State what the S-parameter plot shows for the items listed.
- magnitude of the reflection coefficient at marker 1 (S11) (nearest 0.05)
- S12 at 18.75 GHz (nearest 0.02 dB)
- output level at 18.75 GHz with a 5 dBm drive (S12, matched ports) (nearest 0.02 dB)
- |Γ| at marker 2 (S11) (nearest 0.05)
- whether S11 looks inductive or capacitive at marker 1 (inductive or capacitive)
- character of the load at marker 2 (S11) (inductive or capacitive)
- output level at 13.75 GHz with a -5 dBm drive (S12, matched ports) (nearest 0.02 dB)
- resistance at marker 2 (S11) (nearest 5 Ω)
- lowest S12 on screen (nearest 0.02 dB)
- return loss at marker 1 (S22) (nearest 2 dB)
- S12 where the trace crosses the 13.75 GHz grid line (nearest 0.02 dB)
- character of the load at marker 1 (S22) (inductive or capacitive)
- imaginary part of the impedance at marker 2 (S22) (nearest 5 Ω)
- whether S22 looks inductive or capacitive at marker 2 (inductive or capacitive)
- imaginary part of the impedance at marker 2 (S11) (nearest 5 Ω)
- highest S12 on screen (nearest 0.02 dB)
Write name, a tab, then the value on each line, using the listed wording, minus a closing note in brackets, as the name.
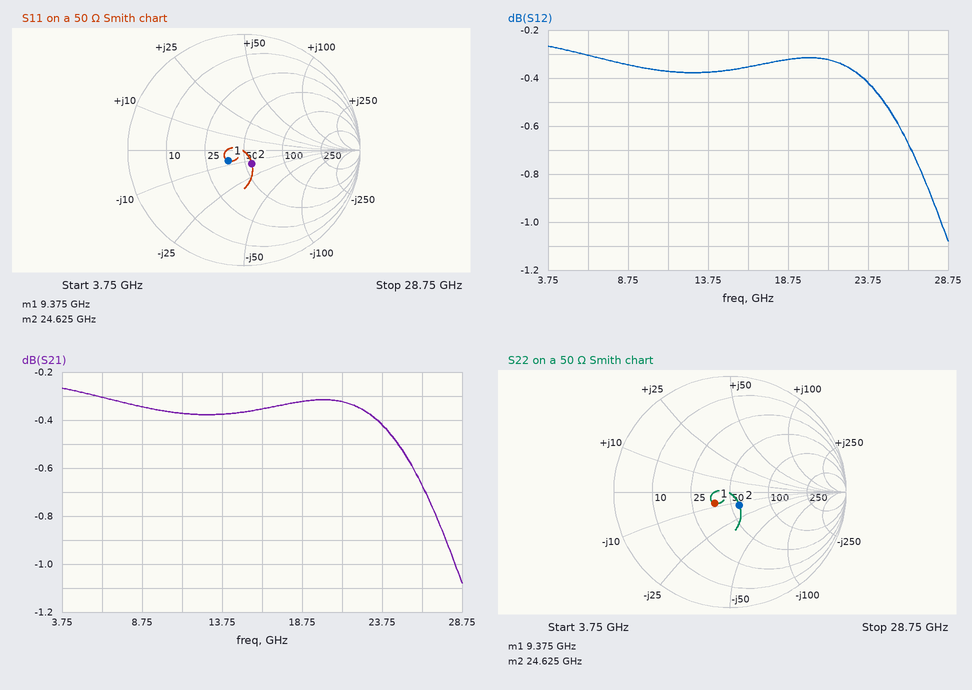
magnitude of the reflection coefficient at marker 1 (S11)	0.15
S12 at 18.75 GHz	-0.32 dB
output level at 18.75 GHz with a 5 dBm drive (S12, matched ports)	4.68 dBm
|Γ| at marker 2 (S11)	0.15
whether S11 looks inductive or capacitive at marker 1	capacitive
character of the load at marker 2 (S11)	capacitive
output level at 13.75 GHz with a -5 dBm drive (S12, matched ports)	-5.38 dBm
resistance at marker 2 (S11)	55 Ω
lowest S12 on screen	-1.08 dB
return loss at marker 1 (S22)	16 dB
S12 where the trace crosses the 13.75 GHz grid line	-0.38 dB
character of the load at marker 1 (S22)	capacitive
imaginary part of the impedance at marker 2 (S22)	-15 Ω
whether S22 looks inductive or capacitive at marker 2	capacitive
imaginary part of the impedance at marker 2 (S11)	-15 Ω
highest S12 on screen	-0.26 dB
